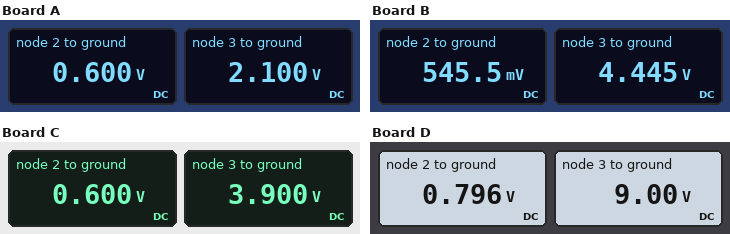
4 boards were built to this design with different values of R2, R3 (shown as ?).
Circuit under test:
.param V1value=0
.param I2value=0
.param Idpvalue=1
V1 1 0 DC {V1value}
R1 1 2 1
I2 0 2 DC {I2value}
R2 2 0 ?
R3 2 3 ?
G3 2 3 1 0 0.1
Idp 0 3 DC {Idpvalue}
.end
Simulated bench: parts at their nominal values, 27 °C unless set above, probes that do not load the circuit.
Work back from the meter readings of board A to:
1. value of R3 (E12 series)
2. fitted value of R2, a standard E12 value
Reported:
1.5 Ω
1.5 Ω
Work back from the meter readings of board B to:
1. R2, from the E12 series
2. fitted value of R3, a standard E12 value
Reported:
1.2 Ω
3.9 Ω
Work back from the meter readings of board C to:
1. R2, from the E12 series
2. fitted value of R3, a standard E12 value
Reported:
1.5 Ω
3.3 Ω
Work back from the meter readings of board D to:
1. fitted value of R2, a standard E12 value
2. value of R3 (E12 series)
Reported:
3.9 Ω
8.2 Ω
